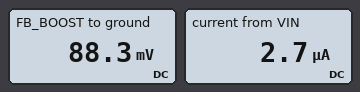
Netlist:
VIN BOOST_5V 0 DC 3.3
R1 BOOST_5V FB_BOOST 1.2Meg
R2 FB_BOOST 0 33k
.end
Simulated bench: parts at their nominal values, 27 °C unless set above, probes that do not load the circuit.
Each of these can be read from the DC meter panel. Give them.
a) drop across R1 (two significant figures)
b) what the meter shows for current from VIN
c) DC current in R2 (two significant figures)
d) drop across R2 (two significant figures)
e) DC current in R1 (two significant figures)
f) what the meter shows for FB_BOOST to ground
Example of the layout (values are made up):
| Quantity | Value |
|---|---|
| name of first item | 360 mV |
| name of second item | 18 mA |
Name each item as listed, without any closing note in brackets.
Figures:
| Quantity | Value |
|---|---|
| drop across R1 | 3.2 V |
| what the meter shows for current from VIN | 2.7 µA |
| DC current in R2 | 2.7 µA |
| drop across R2 | 88 mV |
| DC current in R1 | 2.7 µA |
| what the meter shows for FB_BOOST to ground | 88.3 mV |
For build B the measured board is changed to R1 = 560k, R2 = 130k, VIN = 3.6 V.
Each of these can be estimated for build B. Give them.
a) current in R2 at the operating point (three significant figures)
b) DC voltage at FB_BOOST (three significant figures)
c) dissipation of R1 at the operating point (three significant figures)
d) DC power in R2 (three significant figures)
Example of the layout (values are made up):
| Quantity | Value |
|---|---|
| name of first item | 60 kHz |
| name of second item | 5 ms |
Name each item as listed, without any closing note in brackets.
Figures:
| Quantity | Value |
|---|---|
| current in R2 at the operating point | 5.22 µA |
| DC voltage at FB_BOOST | 678 mV |
| dissipation of R1 at the operating point | 15.2 µW |
| DC power in R2 | 3.54 µW |
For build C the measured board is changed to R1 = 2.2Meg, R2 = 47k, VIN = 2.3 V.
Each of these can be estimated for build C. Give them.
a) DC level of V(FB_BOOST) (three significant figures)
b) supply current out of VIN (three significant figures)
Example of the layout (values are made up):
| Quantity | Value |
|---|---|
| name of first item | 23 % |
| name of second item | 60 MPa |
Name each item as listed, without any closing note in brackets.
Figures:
| Quantity | Value |
|---|---|
| DC level of V(FB_BOOST) | 48.1 mV |
| supply current out of VIN | 1.02 µA |
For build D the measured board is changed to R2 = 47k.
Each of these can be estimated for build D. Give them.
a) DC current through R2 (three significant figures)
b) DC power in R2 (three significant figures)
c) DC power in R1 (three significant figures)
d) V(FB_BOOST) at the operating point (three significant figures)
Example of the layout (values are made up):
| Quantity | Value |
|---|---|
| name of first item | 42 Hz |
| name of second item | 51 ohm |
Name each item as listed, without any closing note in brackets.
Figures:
| Quantity | Value |
|---|---|
| DC current through R2 | 2.65 µA |
| DC power in R2 | 329 nW |
| DC power in R1 | 8.40 µW |
| V(FB_BOOST) at the operating point | 124 mV |
